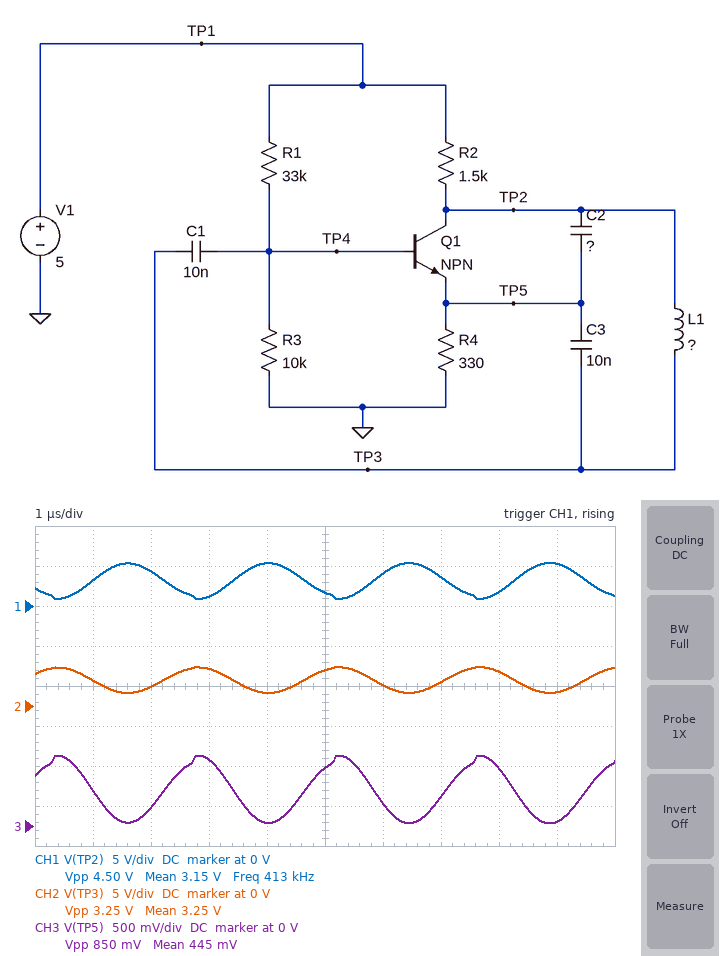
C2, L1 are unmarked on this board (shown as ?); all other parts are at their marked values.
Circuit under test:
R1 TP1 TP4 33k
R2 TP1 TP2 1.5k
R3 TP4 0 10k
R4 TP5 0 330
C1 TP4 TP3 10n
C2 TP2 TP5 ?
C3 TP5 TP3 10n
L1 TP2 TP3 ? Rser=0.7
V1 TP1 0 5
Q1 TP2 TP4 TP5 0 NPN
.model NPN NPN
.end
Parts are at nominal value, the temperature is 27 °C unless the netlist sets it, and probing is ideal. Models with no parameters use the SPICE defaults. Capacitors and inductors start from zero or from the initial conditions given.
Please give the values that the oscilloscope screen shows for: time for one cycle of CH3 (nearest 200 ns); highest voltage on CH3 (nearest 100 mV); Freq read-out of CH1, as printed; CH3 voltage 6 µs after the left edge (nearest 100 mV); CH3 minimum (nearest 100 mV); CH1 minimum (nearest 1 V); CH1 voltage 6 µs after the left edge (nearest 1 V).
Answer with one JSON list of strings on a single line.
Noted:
["2.4 µs", "900 mV", "413 kHz", "300 mV", "0 V", "1 V", "4 V"]
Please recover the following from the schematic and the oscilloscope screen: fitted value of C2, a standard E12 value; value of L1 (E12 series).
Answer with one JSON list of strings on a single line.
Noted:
["4.7 nF", "47 µH"]
